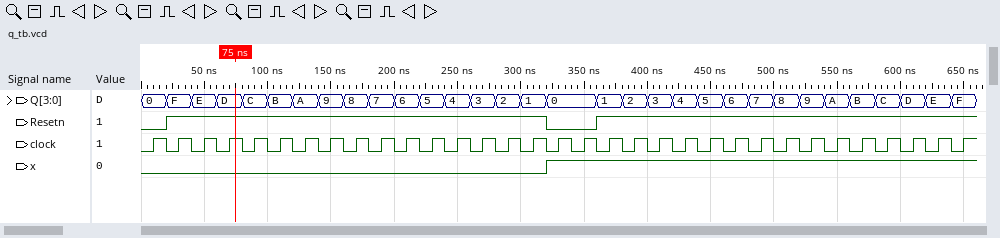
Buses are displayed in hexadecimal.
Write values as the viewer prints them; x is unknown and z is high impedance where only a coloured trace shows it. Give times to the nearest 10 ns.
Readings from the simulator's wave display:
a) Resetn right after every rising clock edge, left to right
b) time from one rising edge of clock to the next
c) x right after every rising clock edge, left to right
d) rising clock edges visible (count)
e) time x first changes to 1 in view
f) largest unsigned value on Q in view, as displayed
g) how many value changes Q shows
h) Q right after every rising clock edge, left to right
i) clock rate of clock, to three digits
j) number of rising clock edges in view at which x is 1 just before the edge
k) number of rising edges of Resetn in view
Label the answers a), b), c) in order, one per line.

a) 0 1 1 1 1 1 1 1 1 1 1 1 1 1 1 1 0 0 1 1 1 1 1 1 1 1 1 1 1 1 1 1 1
b) 20 ns
c) 0 0 0 0 0 0 0 0 0 0 0 0 0 0 0 0 1 1 1 1 1 1 1 1 1 1 1 1 1 1 1 1 1
d) 33
e) 320 ns
f) F
g) 31
h) 0, F, E, D, C, B, A, 9, 8, 7, 6, 5, 4, 3, 2, 1, 0, 0, 1, 2, 3, 4, 5, 6, 7, 8, 9, A, B, C, D, E, F
i) 50.0 MHz
j) 17
k) 2
